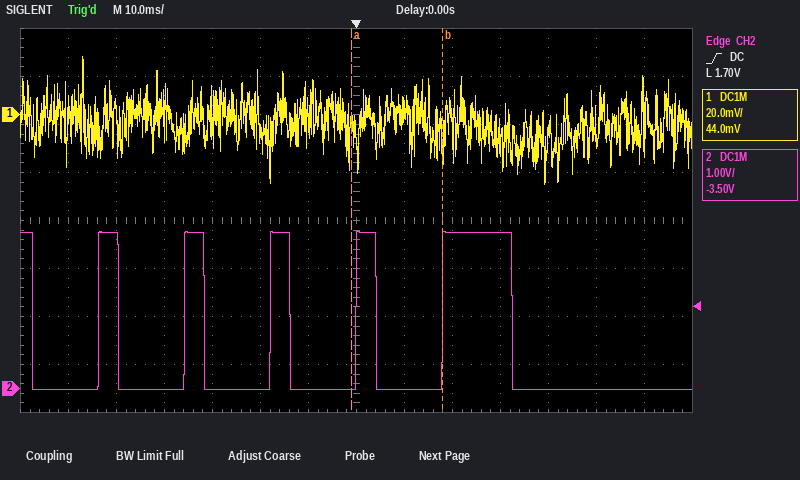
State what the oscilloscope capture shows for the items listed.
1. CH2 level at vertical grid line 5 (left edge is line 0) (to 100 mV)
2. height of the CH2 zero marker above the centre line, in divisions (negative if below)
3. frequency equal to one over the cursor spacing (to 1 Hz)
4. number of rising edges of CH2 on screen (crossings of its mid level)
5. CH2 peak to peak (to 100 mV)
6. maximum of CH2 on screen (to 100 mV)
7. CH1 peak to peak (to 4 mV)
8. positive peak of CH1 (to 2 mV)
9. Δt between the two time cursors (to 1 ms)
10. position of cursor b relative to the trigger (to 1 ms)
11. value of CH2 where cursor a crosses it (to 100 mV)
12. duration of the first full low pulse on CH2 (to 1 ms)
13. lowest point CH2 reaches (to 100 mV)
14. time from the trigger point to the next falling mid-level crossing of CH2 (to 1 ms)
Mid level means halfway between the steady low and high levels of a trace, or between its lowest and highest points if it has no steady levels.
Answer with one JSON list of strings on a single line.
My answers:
["0.0 V", "-3.5 div", "53 Hz", "5", "3.3 V", "3.3 V", "52 mV", "24 mV", "19 ms", "+18 ms", "0.0 V", "14 ms", "0.0 V", "4 ms"]
